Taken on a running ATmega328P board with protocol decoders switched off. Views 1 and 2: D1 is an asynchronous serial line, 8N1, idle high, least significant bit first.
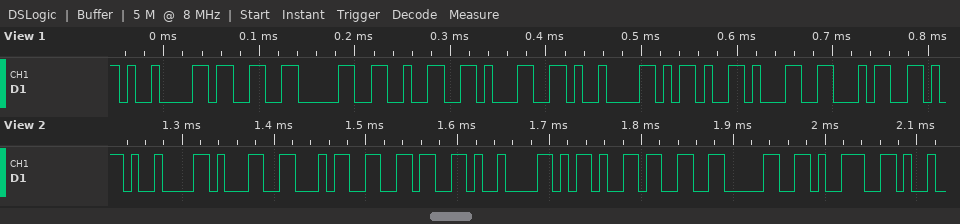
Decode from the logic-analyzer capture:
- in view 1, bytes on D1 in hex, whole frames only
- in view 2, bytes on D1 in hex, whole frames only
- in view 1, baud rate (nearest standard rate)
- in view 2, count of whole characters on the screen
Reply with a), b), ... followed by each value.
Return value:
a) 0x09 0x33 0x30 0x32 0x31 0x09 0x2D 0x31 0x34
b) 09 31 34 36 09 2D 33 30 39
c) 115200 baud
d) 9
